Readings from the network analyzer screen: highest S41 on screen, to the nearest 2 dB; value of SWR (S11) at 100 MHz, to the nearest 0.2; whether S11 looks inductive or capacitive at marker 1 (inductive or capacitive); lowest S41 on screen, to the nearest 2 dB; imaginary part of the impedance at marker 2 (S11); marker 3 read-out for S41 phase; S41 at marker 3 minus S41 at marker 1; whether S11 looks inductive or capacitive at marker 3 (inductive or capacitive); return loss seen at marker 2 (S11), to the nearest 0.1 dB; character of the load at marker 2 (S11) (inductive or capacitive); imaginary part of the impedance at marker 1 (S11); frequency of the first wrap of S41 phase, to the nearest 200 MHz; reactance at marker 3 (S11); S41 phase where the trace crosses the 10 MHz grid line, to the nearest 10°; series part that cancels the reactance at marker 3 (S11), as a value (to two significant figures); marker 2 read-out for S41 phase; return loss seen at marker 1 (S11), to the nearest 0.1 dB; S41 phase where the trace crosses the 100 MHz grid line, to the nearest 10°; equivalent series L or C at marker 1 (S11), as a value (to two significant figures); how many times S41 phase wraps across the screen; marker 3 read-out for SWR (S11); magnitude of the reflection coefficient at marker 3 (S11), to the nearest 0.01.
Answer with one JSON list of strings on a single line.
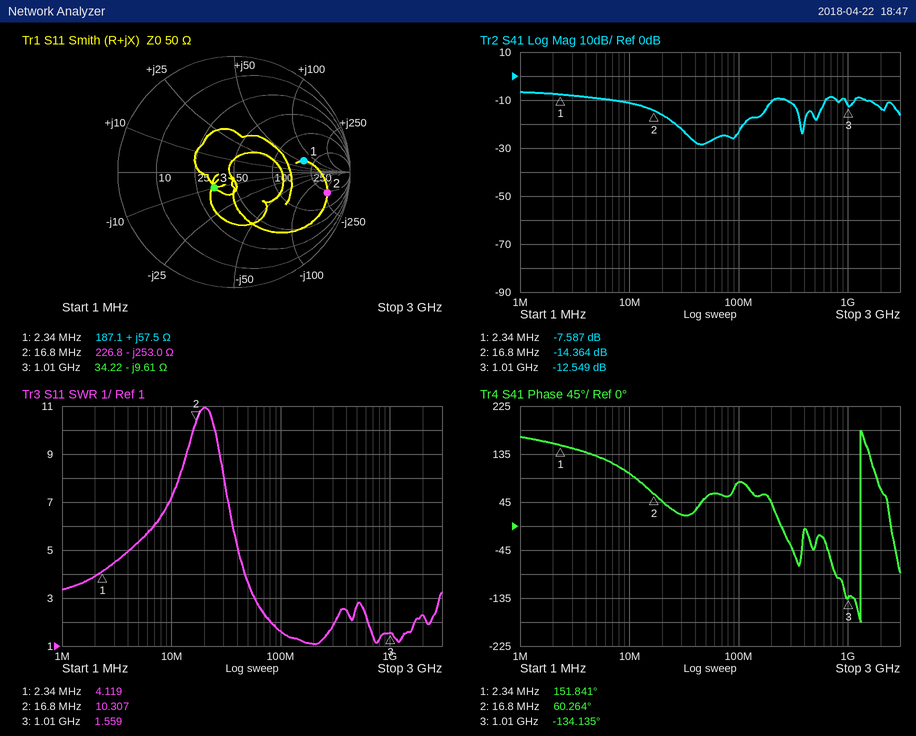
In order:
["-6 dB", "1.6", "inductive", "-28 dB", "-253.0 Ω", "-134.135°", "-4.962 dB", "capacitive", "1.7 dB", "capacitive", "+57.5 Ω", "1.4 GHz", "-9.61 Ω", "100°", "1.5 nH", "60.264°", "4.3 dB", "80°", "3.9 µH", "1", "1.559", "0.22"]
